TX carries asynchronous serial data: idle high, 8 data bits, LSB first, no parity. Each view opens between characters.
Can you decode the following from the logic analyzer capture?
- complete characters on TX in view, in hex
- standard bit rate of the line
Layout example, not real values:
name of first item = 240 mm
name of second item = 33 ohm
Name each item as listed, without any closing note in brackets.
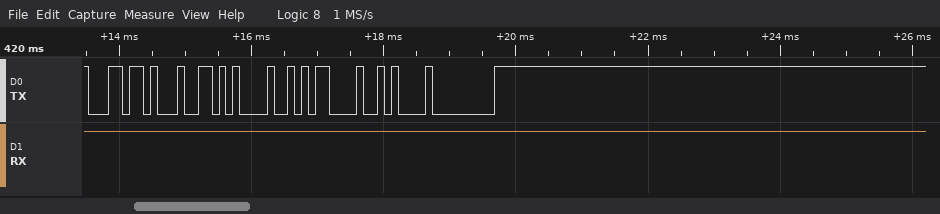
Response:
complete characters on TX in view, in hex = 6C, 64, 21, 0D, 0A, 00
standard bit rate of the line = 9600 baud
